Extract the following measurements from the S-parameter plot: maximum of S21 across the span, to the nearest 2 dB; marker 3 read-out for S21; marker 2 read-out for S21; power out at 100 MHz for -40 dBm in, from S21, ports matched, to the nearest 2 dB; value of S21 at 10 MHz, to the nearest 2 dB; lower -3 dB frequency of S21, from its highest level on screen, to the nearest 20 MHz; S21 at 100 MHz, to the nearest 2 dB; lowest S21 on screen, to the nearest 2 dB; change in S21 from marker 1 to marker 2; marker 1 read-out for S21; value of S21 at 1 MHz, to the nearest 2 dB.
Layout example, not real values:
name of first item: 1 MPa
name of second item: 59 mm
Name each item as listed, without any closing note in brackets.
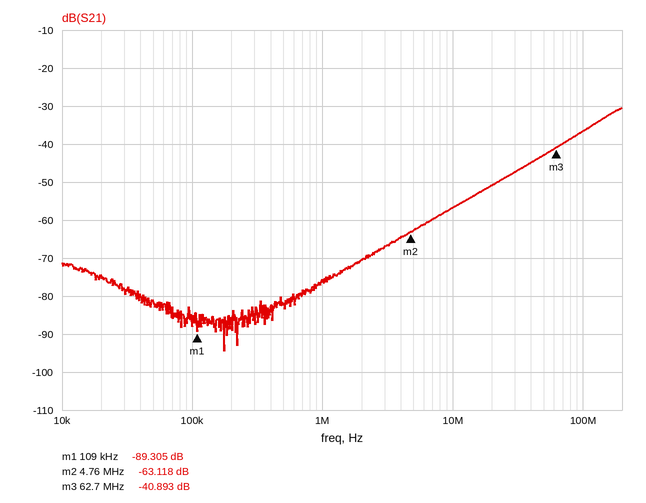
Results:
maximum of S21 across the span, to the nearest 2 dB: -30 dB
marker 3 read-out for S21: -40.893 dB
marker 2 read-out for S21: -63.118 dB
power out at 100 MHz for -40 dBm in, from S21, ports matched, to the nearest 2 dB: -76 dBm
value of S21 at 10 MHz, to the nearest 2 dB: -56 dB
lower -3 dB frequency of S21, from its highest level on screen, to the nearest 20 MHz: 140 MHz
S21 at 100 MHz, to the nearest 2 dB: -36 dB
lowest S21 on screen, to the nearest 2 dB: -94 dB
change in S21 from marker 1 to marker 2: 26.187 dB
marker 1 read-out for S21: -89.305 dB
value of S21 at 1 MHz, to the nearest 2 dB: -76 dB
